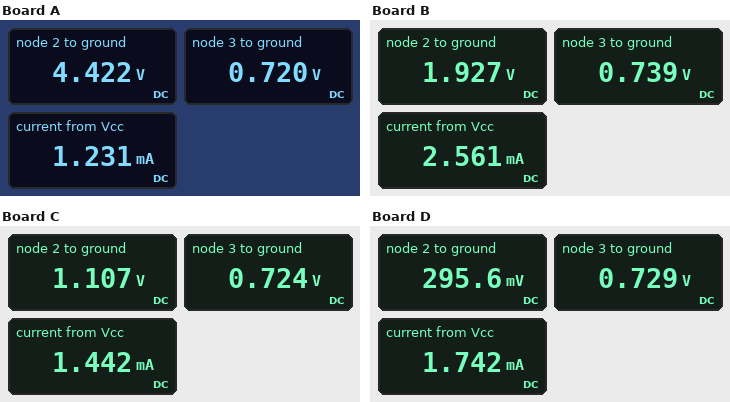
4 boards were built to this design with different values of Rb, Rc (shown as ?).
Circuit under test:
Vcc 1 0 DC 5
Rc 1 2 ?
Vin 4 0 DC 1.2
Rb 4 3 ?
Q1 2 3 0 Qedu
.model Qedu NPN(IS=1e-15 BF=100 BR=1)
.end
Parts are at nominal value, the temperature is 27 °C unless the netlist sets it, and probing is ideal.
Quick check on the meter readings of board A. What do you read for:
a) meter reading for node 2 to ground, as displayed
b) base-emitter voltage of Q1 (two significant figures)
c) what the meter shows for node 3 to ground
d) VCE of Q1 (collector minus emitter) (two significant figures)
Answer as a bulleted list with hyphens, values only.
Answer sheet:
- 4.422 V
- 720 mV
- 0.720 V
- 4.4 V
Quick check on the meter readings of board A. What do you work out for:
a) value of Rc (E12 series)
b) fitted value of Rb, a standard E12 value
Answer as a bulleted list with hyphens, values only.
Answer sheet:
- 470 Ω
- 39 kΩ
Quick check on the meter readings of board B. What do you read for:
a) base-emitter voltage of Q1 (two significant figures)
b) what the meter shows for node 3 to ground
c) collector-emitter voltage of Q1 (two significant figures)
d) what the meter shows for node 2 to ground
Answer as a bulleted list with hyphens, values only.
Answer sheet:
- 740 mV
- 0.739 V
- 1.9 V
- 1.927 V
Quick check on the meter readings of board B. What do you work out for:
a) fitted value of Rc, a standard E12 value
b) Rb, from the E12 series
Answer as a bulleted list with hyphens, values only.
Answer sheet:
- 1.2 kΩ
- 18 kΩ
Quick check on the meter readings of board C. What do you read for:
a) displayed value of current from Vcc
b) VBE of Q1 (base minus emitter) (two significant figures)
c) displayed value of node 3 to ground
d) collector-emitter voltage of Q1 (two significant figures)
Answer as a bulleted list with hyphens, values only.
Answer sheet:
- 1.442 mA
- 720 mV
- 0.724 V
- 1.1 V
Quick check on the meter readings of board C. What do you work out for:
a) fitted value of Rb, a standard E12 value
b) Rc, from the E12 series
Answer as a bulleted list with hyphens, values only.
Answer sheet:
- 33 kΩ
- 2.7 kΩ
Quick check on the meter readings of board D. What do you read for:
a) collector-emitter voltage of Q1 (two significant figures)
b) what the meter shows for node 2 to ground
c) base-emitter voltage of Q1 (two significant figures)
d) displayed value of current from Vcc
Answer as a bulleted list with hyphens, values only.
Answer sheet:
- 300 mV
- 295.6 mV
- 730 mV
- 1.742 mA
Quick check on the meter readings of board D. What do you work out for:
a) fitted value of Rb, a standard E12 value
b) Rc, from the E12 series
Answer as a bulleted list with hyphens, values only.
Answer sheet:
- 27 kΩ
- 2.7 kΩ
